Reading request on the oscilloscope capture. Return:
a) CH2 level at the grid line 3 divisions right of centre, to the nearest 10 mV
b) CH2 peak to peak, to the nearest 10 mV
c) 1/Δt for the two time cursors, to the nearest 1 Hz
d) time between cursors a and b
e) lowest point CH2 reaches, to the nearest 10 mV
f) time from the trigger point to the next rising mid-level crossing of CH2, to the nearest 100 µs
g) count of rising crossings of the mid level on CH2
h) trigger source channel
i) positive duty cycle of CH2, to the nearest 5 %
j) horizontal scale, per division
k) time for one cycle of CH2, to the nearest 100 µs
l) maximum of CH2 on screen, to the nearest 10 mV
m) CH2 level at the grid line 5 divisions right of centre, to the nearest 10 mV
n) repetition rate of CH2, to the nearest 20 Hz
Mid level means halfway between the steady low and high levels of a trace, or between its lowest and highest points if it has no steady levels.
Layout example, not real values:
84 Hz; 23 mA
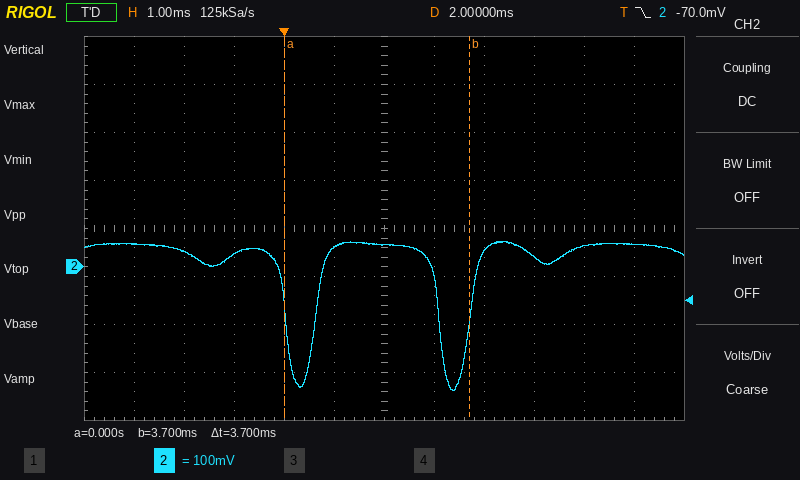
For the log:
20 mV; 310 mV; 270 Hz; 3.7 ms; -260 mV; 600 µs; 2; CH2; 80 %; 1 ms; 3.1 ms; 50 mV; 50 mV; 320 Hz
